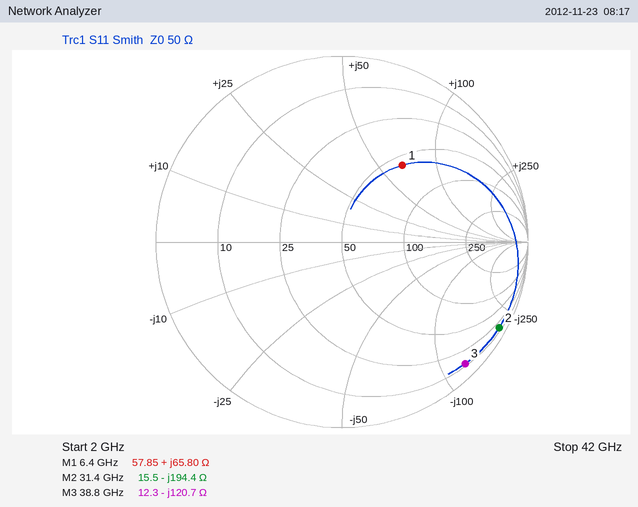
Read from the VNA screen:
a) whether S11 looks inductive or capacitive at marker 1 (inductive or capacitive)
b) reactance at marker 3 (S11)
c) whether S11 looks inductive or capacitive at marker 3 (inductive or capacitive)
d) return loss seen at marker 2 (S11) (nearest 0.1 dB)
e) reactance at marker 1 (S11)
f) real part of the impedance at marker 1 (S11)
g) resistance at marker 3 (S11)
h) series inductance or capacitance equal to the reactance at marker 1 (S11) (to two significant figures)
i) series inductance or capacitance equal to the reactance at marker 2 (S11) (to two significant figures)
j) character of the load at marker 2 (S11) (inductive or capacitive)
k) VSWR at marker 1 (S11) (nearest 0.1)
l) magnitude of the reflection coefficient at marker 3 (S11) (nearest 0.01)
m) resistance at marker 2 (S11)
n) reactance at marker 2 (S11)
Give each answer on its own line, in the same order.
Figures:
inductive
-120.7 Ω
capacitive
0.3 dB
+65.80 Ω
57.85 Ω
12.3 Ω
1.6 nH
26 fF
capacitive
3.2
0.93
15.5 Ω
-194.4 Ω
